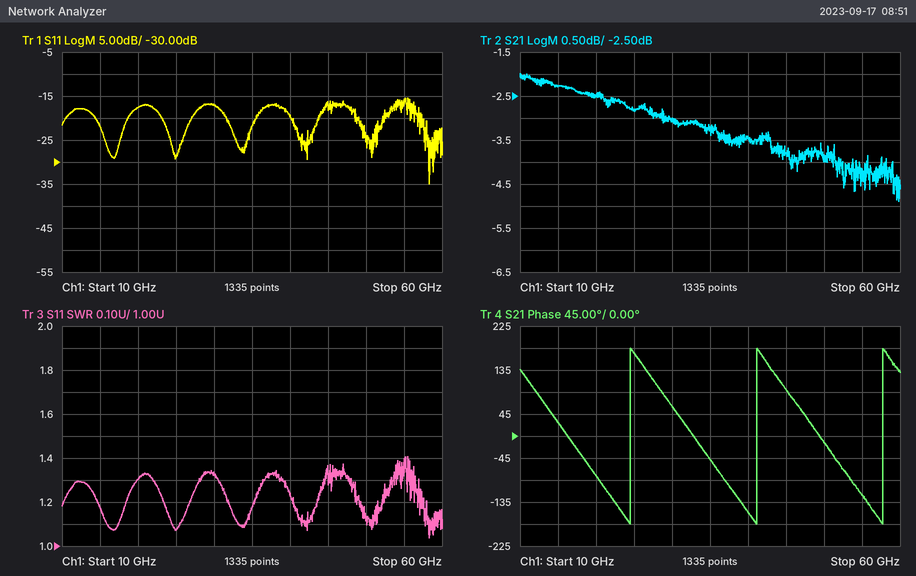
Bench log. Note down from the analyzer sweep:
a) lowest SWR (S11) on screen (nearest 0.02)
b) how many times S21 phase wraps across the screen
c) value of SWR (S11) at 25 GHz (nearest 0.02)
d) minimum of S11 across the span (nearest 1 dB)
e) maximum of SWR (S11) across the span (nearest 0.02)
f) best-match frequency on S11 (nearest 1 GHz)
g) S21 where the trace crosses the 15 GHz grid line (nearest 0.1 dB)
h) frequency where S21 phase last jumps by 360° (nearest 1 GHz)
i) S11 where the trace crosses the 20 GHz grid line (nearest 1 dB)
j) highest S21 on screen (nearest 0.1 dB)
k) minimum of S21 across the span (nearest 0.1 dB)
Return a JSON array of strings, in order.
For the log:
["1.04", "3", "1.08", "-35 dB", "1.40", "58 GHz", "-2.3 dB", "58 GHz", "-18 dB", "-2.0 dB", "-4.9 dB"]
